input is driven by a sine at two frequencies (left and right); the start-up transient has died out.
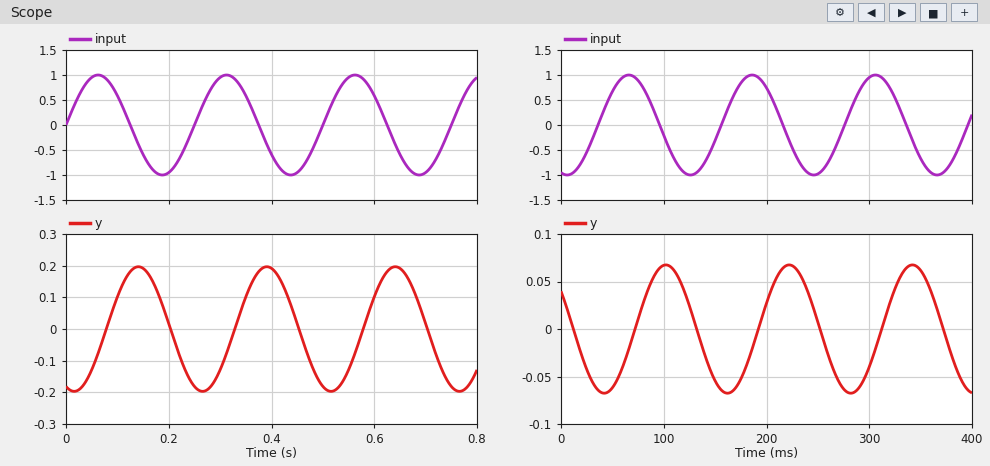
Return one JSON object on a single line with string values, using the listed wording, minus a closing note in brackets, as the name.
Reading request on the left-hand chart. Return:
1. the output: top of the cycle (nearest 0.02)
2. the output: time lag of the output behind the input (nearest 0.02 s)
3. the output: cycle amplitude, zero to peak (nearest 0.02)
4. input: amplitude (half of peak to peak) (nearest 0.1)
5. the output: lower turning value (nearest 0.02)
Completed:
{"the output: top of the cycle": "0.20", "the output: time lag of the output behind the input": "0.08 s", "the output: cycle amplitude, zero to peak": "0.20", "input: amplitude (half of peak to peak)": "1.0", "the output: lower turning value": "-0.20"}
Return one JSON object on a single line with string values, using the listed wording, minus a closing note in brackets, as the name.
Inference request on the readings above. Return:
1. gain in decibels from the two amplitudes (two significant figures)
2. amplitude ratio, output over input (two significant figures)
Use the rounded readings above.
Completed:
{"gain in decibels from the two amplitudes": "-14 dB", "amplitude ratio, output over input": "0.20"}
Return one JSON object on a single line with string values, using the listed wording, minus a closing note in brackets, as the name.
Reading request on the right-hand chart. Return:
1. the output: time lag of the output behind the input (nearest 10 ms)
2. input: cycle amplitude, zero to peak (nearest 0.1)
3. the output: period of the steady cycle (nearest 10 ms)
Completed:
{"the output: time lag of the output behind the input": "40 ms", "input: cycle amplitude, zero to peak": "1.0", "the output: period of the steady cycle": "120 ms"}
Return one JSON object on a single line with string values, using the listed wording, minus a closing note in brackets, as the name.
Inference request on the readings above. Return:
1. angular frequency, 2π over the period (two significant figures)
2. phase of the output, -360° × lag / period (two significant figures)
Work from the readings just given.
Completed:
{"angular frequency, 2π over the period": "0.052 rad/ms", "phase of the output, -360° × lag / period": "-120°"}
